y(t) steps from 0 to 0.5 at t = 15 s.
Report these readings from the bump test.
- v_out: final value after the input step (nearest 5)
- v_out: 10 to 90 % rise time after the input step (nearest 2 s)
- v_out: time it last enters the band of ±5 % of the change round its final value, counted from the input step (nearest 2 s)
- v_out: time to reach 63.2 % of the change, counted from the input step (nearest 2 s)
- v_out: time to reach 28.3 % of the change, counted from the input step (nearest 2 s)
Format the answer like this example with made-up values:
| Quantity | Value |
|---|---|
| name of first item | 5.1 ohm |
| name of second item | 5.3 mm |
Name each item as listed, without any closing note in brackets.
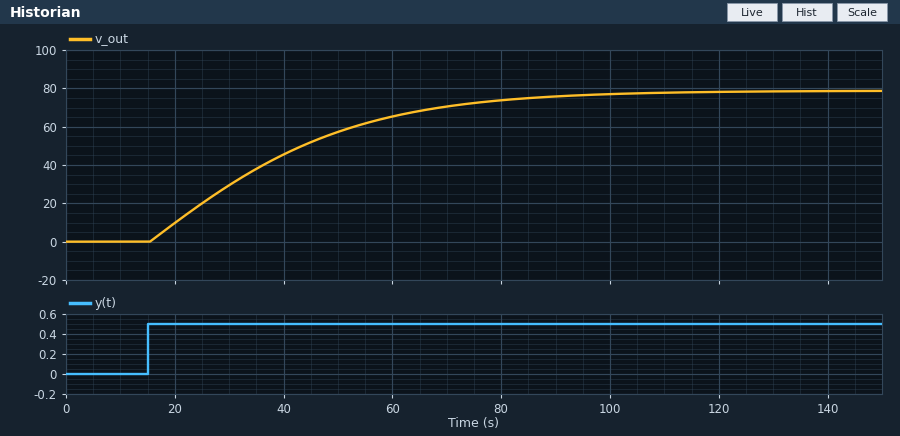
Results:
| Quantity | Value |
|---|---|
| v_out: final value after the input step | 80 |
| v_out: 10 to 90 % rise time after the input step | 52 s |
| v_out: time it last enters the band of ±5 % of the change round its final value, counted from the input step | 70 s |
| v_out: time to reach 63.2 % of the change, counted from the input step | 28 s |
| v_out: time to reach 28.3 % of the change, counted from the input step | 12 s |
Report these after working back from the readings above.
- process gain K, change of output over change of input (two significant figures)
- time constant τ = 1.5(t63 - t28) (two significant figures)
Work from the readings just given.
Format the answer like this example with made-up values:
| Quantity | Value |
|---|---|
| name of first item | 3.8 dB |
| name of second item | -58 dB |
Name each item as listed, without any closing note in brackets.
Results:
| Quantity | Value |
|---|---|
| process gain K, change of output over change of input | 160 |
| time constant τ = 1.5(t63 - t28) | 24 s |
